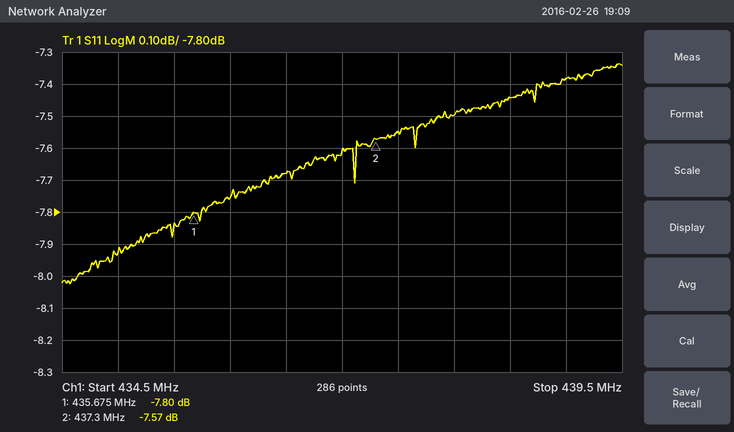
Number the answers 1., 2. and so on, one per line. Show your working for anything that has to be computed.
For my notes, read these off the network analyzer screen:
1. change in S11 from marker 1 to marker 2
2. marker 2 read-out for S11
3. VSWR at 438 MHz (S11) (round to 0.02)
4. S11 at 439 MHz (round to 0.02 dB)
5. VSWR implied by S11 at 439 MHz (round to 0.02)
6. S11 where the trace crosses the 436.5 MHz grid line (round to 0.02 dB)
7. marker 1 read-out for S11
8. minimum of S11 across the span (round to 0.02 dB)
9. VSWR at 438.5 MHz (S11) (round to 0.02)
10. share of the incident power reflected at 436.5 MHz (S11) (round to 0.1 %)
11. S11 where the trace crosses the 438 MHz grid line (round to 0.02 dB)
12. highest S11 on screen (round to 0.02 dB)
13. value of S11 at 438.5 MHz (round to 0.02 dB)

1. -7.57 − (-7.8) = 0.23 dB
2. -7.57 dB
3. |Γ| = 10^(-7.5/20) = 0.4217; VSWR = (1 + 0.4217)/(1 − 0.4217) ≈ 2.46
4. -7.38 dB
5. |Γ| = 10^(-7.38/20) = 0.4276; VSWR = (1 + 0.4276)/(1 − 0.4276) ≈ 2.49, so 2.50 to the nearest 0.02
6. -7.68 dB
7. -7.80 dB
8. -8.02 dB
9. |Γ| = 10^(-7.44/20) = 0.4246; VSWR = (1 + 0.4246)/(1 − 0.4246) ≈ 2.48
10. 10^(-7.68/10) ≈ 17.1 %
11. -7.50 dB
12. -7.34 dB
13. -7.44 dB
